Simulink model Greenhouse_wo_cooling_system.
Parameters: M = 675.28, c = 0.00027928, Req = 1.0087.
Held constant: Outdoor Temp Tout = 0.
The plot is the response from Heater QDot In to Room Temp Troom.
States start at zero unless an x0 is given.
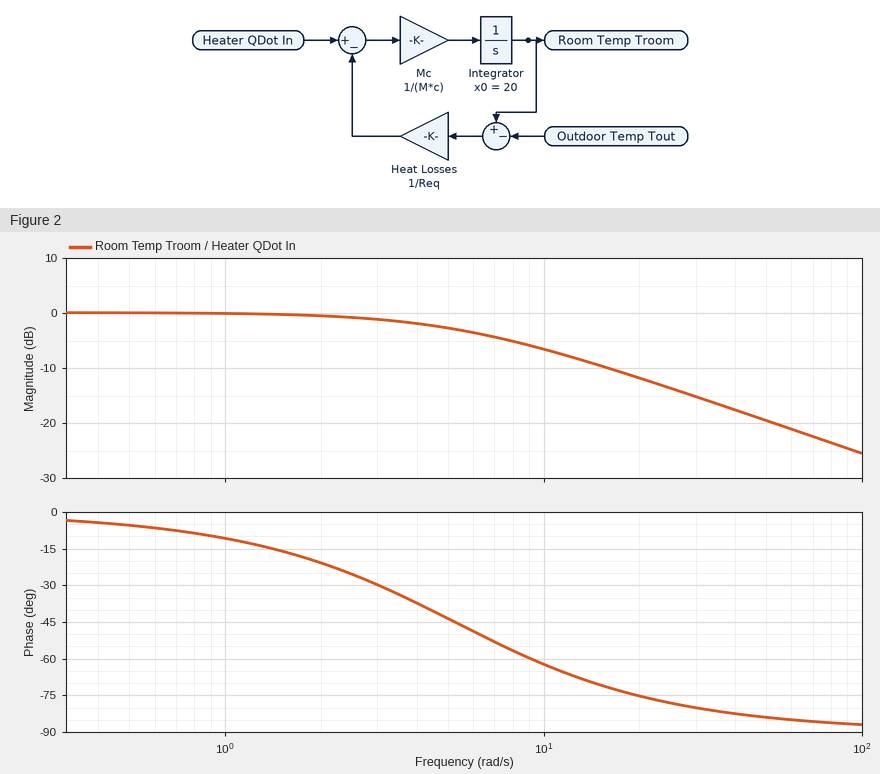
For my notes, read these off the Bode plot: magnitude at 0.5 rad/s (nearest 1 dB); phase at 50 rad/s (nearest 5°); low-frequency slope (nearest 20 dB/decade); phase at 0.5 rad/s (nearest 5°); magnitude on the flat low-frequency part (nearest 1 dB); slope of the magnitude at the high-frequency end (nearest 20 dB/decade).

0 dB
-85°
0 dB/decade
-5°
0 dB
-20 dB/decade
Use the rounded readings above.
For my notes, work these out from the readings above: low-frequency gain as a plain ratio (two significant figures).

1.0
